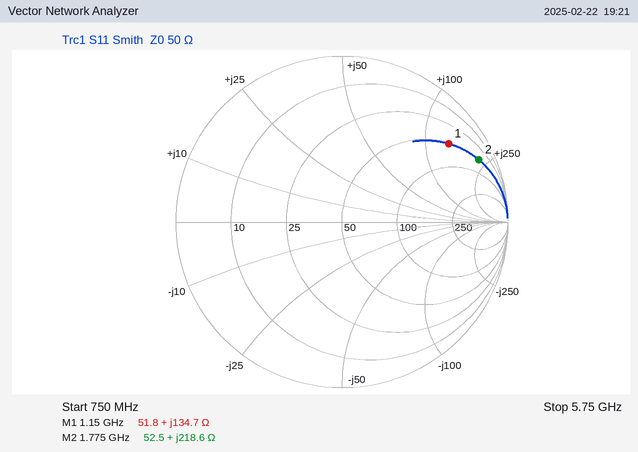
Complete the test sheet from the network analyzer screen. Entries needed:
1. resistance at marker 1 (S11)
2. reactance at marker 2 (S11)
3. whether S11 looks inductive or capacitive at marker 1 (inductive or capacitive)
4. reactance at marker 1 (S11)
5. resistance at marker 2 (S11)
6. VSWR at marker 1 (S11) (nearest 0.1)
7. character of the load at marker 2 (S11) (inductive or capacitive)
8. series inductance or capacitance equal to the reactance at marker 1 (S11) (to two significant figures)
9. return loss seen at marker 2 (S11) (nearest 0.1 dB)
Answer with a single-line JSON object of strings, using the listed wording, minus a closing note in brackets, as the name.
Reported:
{"resistance at marker 1": "51.8 Ω", "reactance at marker 2": "+218.6 Ω", "whether S11 looks inductive or capacitive at marker 1": "inductive", "reactance at marker 1": "+134.7 Ω", "resistance at marker 2": "52.5 Ω", "VSWR at marker 1 (S11)": "8.9", "character of the load at marker 2 (S11)": "inductive", "series inductance or capacitance equal to the reactance at marker 1 (S11)": "19 nH", "return loss seen at marker 2 (S11)": "0.9 dB"}
